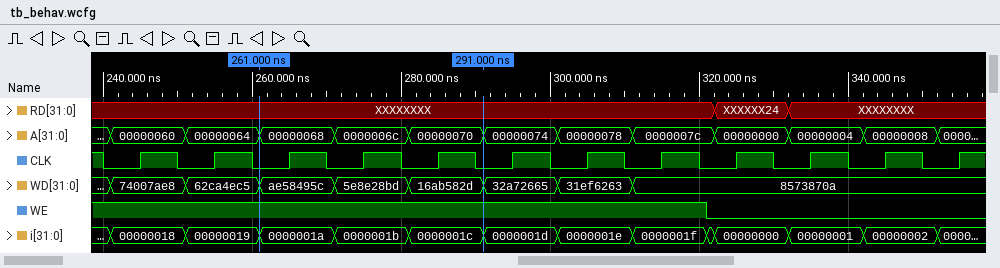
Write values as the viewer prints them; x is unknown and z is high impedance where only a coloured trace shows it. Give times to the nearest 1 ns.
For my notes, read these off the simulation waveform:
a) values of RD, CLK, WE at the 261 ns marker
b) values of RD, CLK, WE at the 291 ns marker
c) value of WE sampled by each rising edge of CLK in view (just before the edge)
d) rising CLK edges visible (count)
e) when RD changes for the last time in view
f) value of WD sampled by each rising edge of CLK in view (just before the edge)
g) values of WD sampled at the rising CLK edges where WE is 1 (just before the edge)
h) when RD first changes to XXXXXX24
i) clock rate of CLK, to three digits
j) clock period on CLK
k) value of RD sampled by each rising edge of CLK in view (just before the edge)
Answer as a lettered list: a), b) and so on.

a) RD=XXXXXXXX, CLK=0, WE=1
b) RD=XXXXXXXX, CLK=0, WE=1
c) 1 1 1 1 1 1 1 1 0 0 0 0
d) 12
e) 332 ns
f) 74007ae8, 62ca4ec5, ae58495c, 5e8e28bd, 16ab582d, 32a72665, 31ef6263, 8573870a, 8573870a, 8573870a, 8573870a, 8573870a
g) 74007ae8, 62ca4ec5, ae58495c, 5e8e28bd, 16ab582d, 32a72665, 31ef6263, 8573870a
h) 322 ns
i) 100 MHz
j) 10 ns
k) XXXXXXXX, XXXXXXXX, XXXXXXXX, XXXXXXXX, XXXXXXXX, XXXXXXXX, XXXXXXXX, XXXXXXXX, XXXXXX24, XXXXXXXX, XXXXXXXX, XXXXXXXX
